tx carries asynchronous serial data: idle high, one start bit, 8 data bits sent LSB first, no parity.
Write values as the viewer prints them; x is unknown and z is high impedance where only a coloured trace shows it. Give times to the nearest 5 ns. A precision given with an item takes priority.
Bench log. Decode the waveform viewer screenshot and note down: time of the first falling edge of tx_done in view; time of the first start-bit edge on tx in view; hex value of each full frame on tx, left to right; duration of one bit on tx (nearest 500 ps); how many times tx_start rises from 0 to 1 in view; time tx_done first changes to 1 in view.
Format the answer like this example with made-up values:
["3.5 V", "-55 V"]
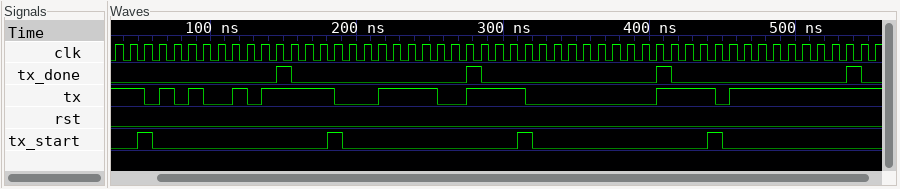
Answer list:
["155 ns", "55 ns", "A5, 3C, 00, FF", "10000 ps", "4", "145 ns"]
